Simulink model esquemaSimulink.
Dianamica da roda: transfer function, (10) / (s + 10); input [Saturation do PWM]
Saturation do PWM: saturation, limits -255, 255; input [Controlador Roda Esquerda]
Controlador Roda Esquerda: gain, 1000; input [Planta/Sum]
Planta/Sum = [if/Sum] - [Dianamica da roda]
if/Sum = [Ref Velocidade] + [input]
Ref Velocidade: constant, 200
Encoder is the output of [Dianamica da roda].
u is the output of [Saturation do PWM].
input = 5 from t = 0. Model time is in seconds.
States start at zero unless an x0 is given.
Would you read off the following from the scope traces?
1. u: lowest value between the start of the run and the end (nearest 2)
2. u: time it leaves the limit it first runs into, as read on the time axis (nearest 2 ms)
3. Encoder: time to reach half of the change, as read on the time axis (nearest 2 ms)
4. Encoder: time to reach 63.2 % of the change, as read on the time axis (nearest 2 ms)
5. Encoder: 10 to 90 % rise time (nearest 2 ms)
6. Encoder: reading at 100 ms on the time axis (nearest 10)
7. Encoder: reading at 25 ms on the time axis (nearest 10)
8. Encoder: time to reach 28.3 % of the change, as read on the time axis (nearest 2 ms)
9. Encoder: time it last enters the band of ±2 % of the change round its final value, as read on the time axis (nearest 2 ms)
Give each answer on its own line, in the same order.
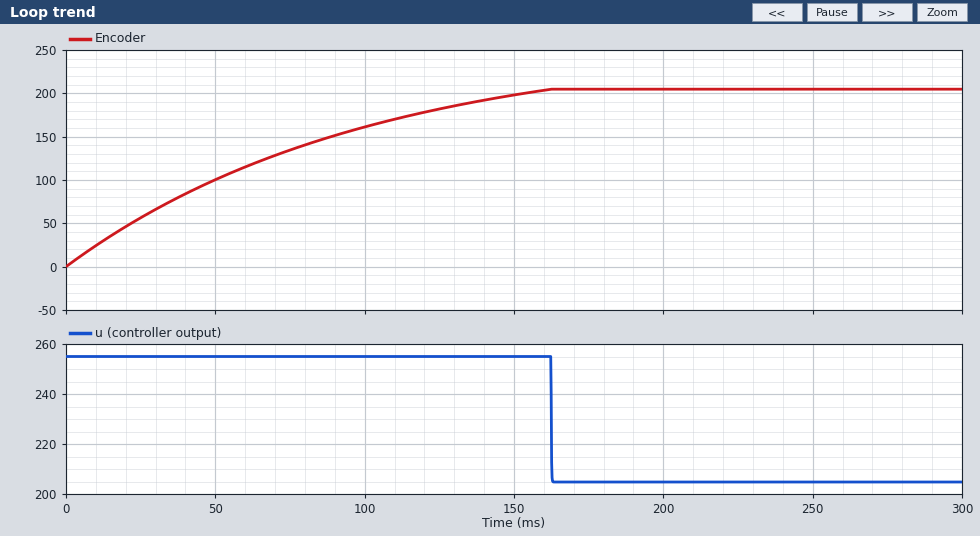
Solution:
204
162 ms
52 ms
70 ms
120 ms
160
60
26 ms
154 ms
